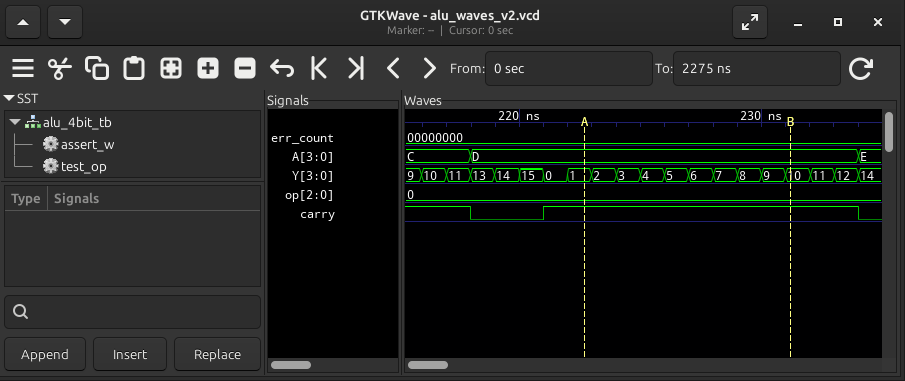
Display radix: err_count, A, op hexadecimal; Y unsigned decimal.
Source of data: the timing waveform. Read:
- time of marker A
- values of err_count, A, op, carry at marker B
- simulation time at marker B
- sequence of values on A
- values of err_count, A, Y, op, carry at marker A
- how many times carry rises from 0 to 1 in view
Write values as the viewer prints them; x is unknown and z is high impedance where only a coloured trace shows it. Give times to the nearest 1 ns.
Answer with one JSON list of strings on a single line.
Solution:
["223 ns", "err_count=00000000, A=D, op=0, carry=1", "231 ns", "C, D, E", "err_count=00000000, A=D, Y=1, op=0, carry=1", "1"]
